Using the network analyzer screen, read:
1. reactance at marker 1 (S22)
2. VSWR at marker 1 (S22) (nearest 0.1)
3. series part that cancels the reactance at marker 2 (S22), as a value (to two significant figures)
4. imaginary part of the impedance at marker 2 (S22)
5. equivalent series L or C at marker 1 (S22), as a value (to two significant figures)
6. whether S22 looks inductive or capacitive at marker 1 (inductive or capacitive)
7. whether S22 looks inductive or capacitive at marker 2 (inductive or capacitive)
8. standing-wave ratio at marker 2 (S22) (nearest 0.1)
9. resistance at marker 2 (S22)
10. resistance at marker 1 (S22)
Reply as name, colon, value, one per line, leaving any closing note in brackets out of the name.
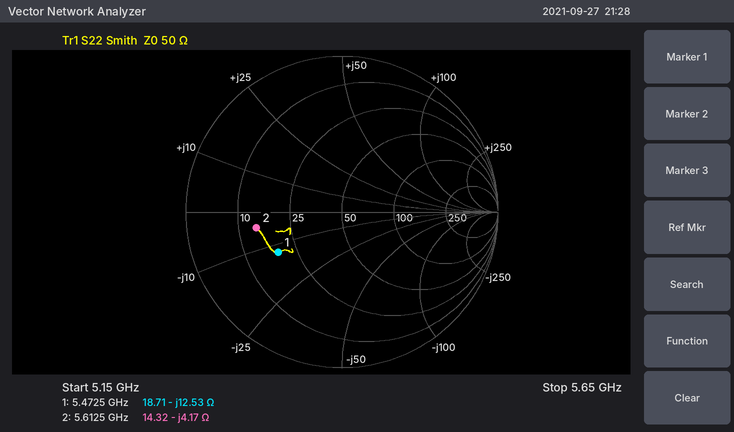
reactance at marker 1: -12.53 Ω
VSWR at marker 1 (S22): 2.9
series part that cancels the reactance at marker 2 (S22), as a value: 120 pH
imaginary part of the impedance at marker 2: -4.17 Ω
equivalent series L or C at marker 1 (S22), as a value: 2.3 pF
whether S22 looks inductive or capacitive at marker 1: capacitive
whether S22 looks inductive or capacitive at marker 2: capacitive
standing-wave ratio at marker 2 (S22): 3.5
resistance at marker 2: 14.32 Ω
resistance at marker 1: 18.71 Ω
